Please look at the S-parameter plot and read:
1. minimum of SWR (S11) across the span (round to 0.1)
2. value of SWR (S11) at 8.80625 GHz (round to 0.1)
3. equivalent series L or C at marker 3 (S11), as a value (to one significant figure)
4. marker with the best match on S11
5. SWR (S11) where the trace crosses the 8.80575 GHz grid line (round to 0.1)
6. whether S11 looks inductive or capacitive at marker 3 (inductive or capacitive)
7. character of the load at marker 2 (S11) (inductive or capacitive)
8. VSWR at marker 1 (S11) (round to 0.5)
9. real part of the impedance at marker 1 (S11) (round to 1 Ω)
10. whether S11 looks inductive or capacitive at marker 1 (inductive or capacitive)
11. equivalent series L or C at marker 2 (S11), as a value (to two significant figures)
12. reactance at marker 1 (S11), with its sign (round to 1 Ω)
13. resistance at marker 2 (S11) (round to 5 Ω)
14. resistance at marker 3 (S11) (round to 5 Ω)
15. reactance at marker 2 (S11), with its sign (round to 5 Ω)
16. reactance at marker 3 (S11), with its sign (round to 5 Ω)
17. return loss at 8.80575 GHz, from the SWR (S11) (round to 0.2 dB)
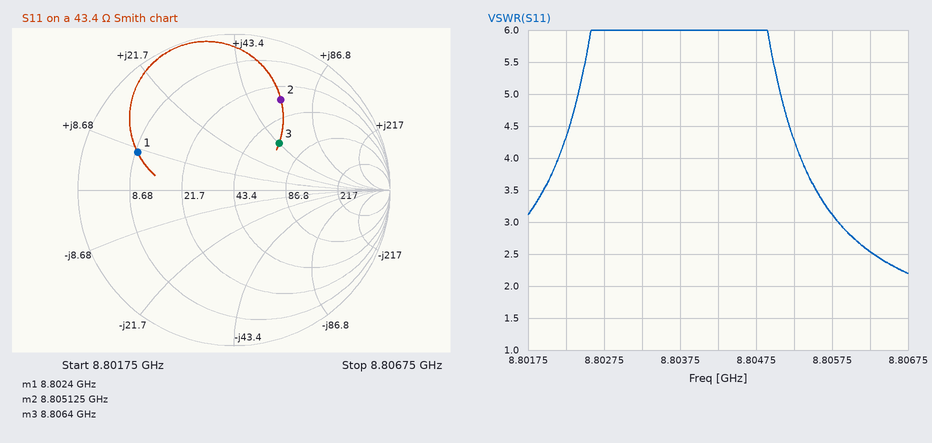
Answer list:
2.2
2.5
800 pH
marker 3
3.1
inductive
inductive
5.0
9 Ω
inductive
1.1 nH
+8 Ω
30 Ω
60 Ω
+60 Ω
+45 Ω
5.8 dB
